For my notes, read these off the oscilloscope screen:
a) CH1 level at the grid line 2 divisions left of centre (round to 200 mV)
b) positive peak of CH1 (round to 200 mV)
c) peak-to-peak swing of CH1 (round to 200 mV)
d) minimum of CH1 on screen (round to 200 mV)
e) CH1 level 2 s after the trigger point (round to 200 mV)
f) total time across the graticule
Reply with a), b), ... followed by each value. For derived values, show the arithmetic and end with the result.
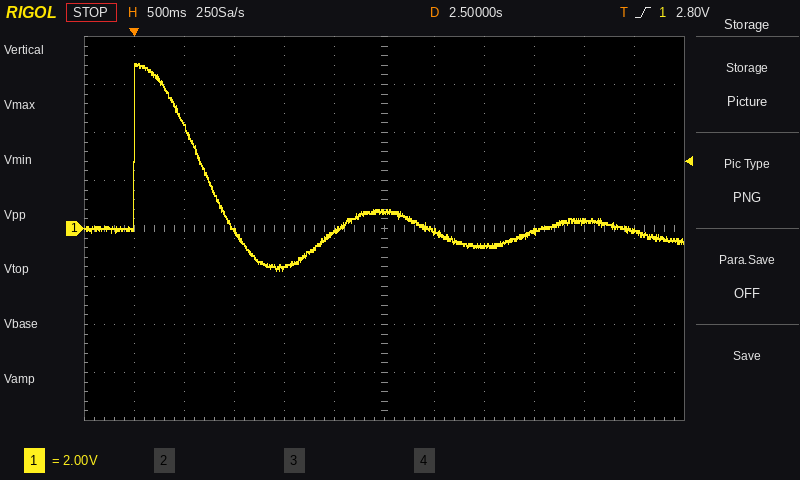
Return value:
a) -1.6 V
b) 6.8 V
c) 6.8 V − (-1.8 V) = 8.6 V
d) -1.8 V
e) -200 mV
f) 6 s
